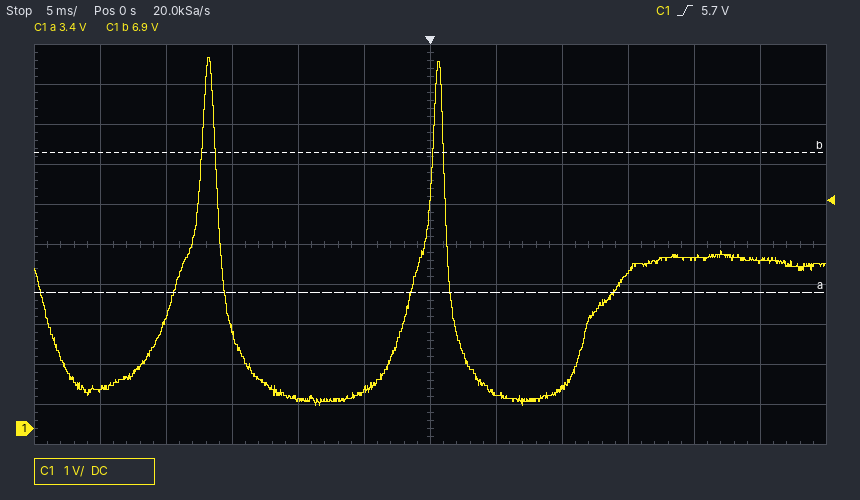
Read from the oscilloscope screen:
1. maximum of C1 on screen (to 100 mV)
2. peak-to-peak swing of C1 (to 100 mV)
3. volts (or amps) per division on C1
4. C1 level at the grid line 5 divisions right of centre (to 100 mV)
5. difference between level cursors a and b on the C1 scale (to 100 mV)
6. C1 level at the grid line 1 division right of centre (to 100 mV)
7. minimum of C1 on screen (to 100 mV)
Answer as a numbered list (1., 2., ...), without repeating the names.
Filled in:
1. 9.3 V
2. 8.7 V
3. 1 V
4. 4.2 V
5. 3.5 V
6. 900 mV
7. 600 mV
